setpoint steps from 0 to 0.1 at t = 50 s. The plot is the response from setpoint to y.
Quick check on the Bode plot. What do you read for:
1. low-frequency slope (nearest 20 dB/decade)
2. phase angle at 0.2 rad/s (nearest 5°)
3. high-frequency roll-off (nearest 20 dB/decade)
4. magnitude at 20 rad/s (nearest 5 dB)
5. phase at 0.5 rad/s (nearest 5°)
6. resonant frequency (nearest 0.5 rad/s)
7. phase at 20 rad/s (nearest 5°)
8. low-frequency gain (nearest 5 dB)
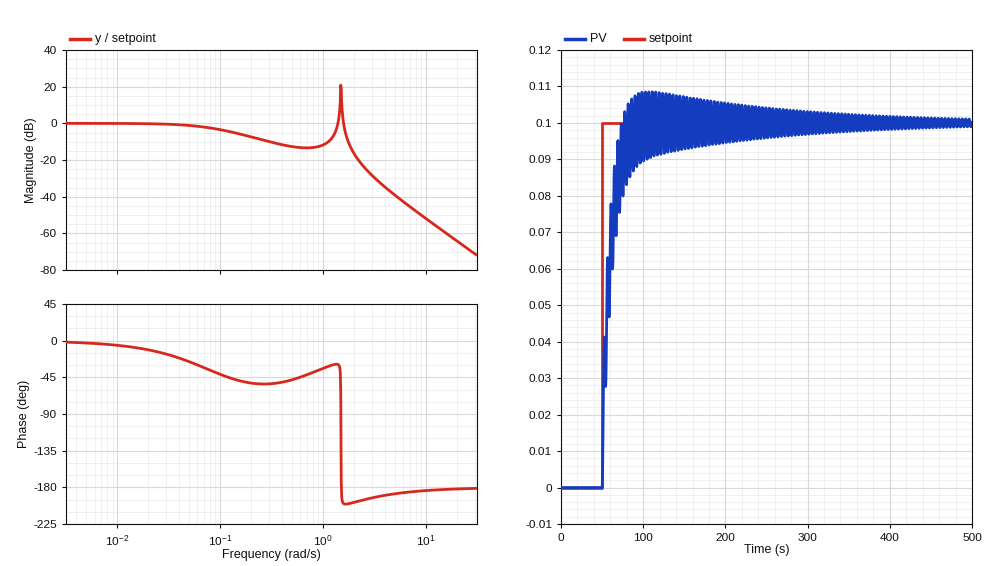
0 dB/decade
-50°
-40 dB/decade
-65 dB
-50°
1.5 rad/s
-180°
0 dB
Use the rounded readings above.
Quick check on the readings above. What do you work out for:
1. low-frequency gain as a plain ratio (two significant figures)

1.0
